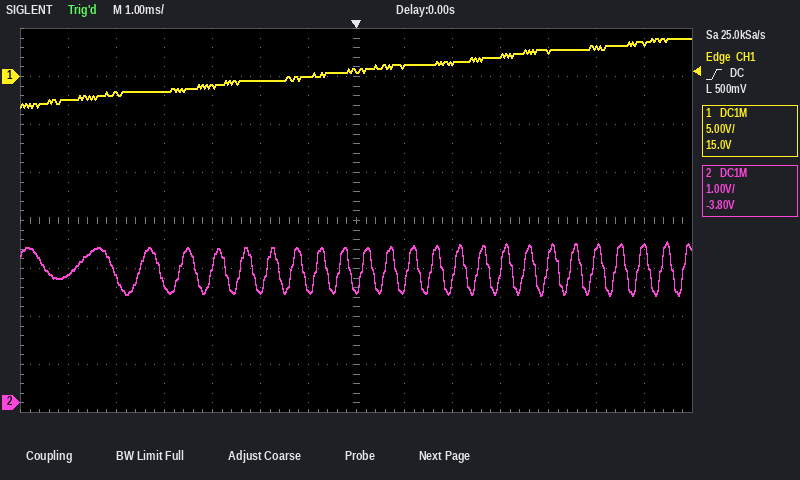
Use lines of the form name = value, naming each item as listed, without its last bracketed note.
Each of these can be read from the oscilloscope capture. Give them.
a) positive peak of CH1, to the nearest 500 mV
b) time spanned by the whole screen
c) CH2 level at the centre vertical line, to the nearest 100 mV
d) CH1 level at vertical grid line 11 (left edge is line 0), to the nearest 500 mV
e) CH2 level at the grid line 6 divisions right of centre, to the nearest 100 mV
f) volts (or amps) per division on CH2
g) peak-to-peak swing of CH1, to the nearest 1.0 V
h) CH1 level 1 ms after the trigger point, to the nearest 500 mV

positive peak of CH1, to the nearest 500 mV = 4.0 V
time spanned by the whole screen = 14 ms
CH2 level at the centre vertical line, to the nearest 100 mV = 2.3 V
CH1 level at vertical grid line 11 (left edge is line 0), to the nearest 500 mV = 2.5 V
CH2 level at the grid line 6 divisions right of centre, to the nearest 100 mV = 3.3 V
volts (or amps) per division on CH2 = 1 V
peak-to-peak swing of CH1, to the nearest 1.0 V = 7.0 V
CH1 level 1 ms after the trigger point, to the nearest 500 mV = 1.0 V
